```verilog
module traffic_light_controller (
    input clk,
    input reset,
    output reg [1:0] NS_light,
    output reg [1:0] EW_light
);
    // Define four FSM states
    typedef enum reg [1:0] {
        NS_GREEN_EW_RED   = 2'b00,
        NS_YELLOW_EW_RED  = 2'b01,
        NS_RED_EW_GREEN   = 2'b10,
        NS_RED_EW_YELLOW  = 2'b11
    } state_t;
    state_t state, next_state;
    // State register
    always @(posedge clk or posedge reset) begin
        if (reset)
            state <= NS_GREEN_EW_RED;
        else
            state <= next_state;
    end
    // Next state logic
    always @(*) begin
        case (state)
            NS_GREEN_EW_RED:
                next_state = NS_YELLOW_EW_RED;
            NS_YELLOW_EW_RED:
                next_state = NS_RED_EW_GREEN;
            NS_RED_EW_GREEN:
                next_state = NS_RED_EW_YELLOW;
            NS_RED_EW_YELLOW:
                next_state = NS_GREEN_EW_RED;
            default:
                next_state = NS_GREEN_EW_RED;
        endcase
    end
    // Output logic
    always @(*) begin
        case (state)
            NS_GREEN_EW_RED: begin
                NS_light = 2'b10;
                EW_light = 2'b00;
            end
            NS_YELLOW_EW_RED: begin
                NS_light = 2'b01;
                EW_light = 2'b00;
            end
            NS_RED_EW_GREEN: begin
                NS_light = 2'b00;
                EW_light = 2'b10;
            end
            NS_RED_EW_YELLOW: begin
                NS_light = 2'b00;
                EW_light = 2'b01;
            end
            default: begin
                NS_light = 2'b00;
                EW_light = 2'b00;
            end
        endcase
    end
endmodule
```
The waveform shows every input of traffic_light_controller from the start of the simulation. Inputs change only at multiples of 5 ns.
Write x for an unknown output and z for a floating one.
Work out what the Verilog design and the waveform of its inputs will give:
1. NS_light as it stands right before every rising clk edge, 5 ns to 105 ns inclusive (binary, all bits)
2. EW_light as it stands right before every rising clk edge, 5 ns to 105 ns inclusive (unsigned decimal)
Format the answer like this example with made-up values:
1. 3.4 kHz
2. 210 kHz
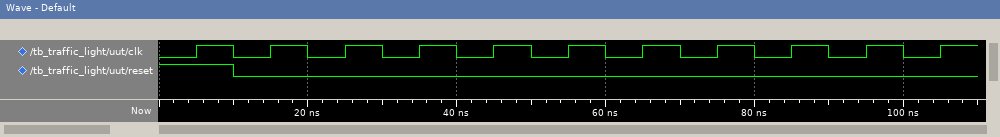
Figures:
1. 10, 10, 01, 00, 00, 10, 01, 00, 00, 10, 01
2. 0, 0, 0, 2, 1, 0, 0, 2, 1, 0, 0
